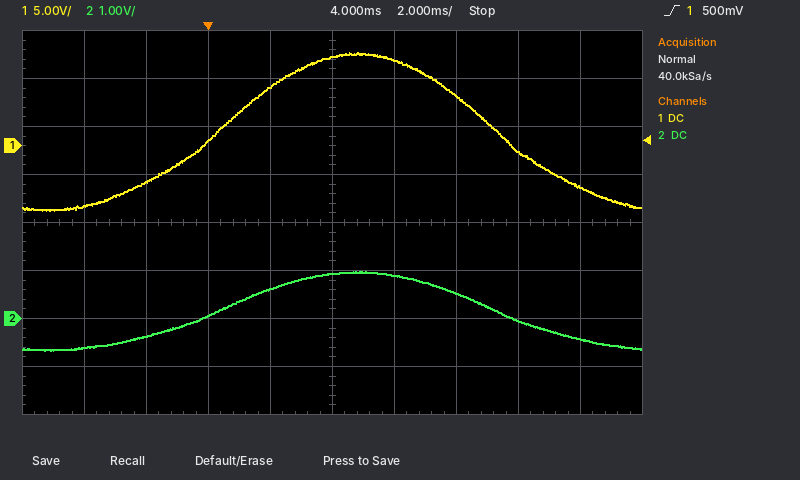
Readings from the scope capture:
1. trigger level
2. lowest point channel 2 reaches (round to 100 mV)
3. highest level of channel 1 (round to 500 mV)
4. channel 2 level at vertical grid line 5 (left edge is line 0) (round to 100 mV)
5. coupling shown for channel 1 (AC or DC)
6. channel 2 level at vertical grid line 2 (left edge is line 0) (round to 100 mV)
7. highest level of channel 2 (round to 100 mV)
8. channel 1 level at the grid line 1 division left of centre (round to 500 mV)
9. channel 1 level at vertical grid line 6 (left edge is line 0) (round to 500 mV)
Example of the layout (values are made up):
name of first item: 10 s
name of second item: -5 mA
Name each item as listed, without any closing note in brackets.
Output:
trigger level: 500 mV
lowest point channel 2 reaches: -700 mV
highest level of channel 1: 9.5 V
channel 2 level at vertical grid line 5 (left edge is line 0): 900 mV
coupling shown for channel 1: DC
channel 2 level at vertical grid line 2 (left edge is line 0): -400 mV
highest level of channel 2: 1.0 V
channel 1 level at the grid line 1 division left of centre: 6.0 V
channel 1 level at vertical grid line 6 (left edge is line 0): 9.0 V
